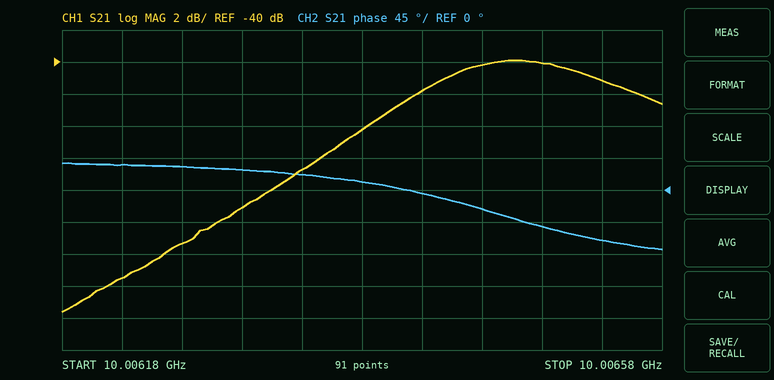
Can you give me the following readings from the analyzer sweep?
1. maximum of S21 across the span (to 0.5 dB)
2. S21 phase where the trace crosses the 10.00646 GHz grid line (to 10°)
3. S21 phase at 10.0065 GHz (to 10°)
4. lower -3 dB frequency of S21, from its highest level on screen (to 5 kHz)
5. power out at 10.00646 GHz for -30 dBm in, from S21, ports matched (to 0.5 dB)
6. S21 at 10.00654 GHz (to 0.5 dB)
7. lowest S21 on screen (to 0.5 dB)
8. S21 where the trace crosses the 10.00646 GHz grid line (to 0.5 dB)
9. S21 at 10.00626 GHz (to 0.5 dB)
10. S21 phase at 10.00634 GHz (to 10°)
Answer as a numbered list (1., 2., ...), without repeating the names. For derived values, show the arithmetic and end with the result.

1. -40.0 dB
2. -30°
3. -50°
4. 10.006400 GHz
5. -30 dBm + (-40.0 dB) = -70.0 dBm
6. -41.0 dB
7. -55.5 dB
8. -40.0 dB
9. -51.5 dB
10. 20°
